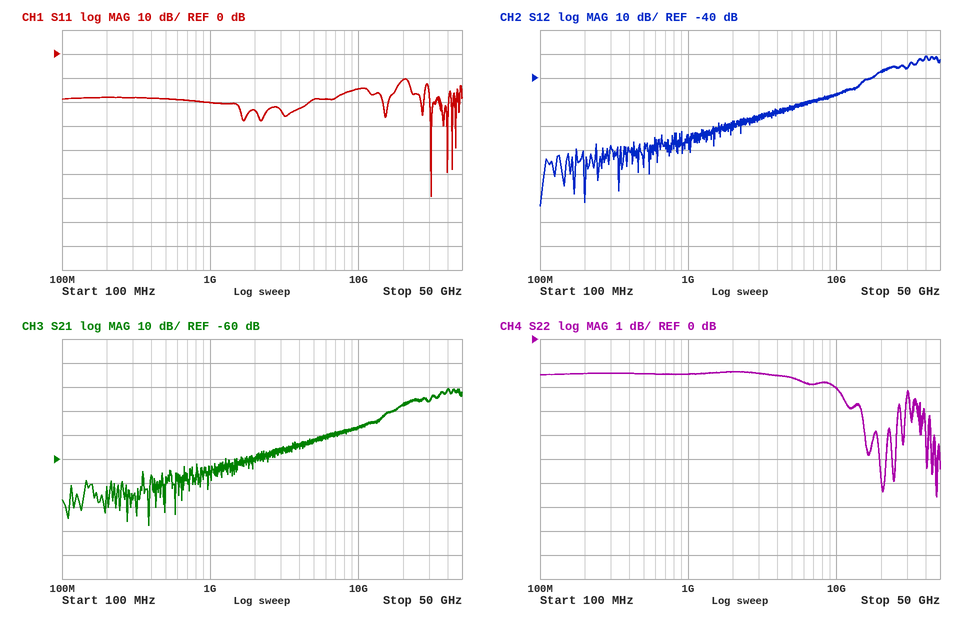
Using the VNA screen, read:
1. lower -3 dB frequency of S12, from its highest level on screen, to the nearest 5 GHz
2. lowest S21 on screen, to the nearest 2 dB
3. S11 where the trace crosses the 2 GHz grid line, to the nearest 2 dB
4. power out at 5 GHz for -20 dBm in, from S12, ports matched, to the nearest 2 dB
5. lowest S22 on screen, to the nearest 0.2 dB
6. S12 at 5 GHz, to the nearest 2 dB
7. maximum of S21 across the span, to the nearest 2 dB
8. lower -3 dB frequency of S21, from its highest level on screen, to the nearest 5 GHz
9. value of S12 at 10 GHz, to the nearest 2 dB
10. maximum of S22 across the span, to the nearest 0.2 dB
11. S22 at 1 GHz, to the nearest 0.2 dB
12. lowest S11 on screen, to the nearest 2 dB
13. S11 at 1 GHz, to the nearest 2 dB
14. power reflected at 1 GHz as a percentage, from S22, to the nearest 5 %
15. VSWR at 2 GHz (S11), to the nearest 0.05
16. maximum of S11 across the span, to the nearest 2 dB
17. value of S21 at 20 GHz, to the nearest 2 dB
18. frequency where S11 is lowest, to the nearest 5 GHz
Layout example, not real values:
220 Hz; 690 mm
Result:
35 GHz; -88 dB; -24 dB; -72 dBm; -6.6 dB; -52 dB; -30 dB; 35 GHz; -46 dB; -1.4 dB; -1.4 dB; -60 dB; -20 dB; 70 %; 1.15; -10 dB; -38 dB; 30 GHz
